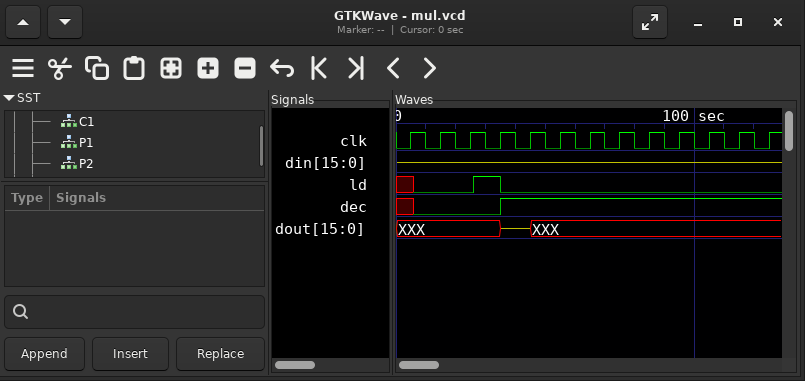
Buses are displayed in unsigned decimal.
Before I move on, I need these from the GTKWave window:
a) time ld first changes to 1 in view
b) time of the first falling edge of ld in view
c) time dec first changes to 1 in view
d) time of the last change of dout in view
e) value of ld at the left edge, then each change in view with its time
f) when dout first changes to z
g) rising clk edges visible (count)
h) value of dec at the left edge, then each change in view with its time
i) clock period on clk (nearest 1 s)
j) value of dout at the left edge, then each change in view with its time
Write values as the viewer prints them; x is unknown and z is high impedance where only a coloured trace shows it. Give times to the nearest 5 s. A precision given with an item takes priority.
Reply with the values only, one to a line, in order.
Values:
25 s
35 s
35 s
45 s
x, 0 at 5 s, 1 at 25 s, 0 at 35 s
35 s
13
x, 0 at 5 s, 1 at 35 s
10 s
XXX, z at 35 s, XXX at 45 s
